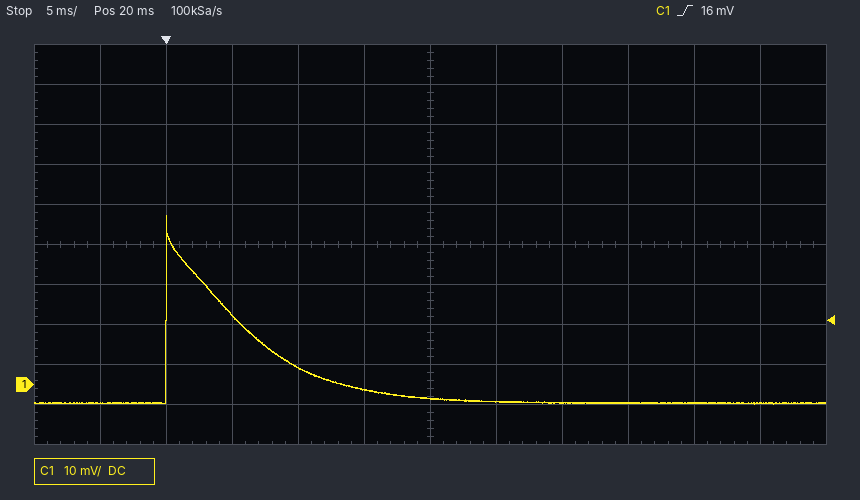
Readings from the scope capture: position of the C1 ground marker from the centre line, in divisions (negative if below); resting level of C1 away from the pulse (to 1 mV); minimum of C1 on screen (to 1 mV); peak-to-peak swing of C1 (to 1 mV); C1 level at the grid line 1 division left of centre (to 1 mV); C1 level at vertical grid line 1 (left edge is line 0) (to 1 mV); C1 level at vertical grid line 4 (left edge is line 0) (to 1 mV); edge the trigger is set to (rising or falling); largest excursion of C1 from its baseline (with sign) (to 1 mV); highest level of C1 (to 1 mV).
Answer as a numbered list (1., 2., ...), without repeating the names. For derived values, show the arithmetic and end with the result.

1. -3.5 div
2. -5 mV
3. -5 mV
4. 42 mV − (-5 mV) = 47 mV
5. -1 mV
6. -5 mV
7. 4 mV
8. rising
9. 42 mV − (-5 mV) = +47 mV
10. 42 mV
